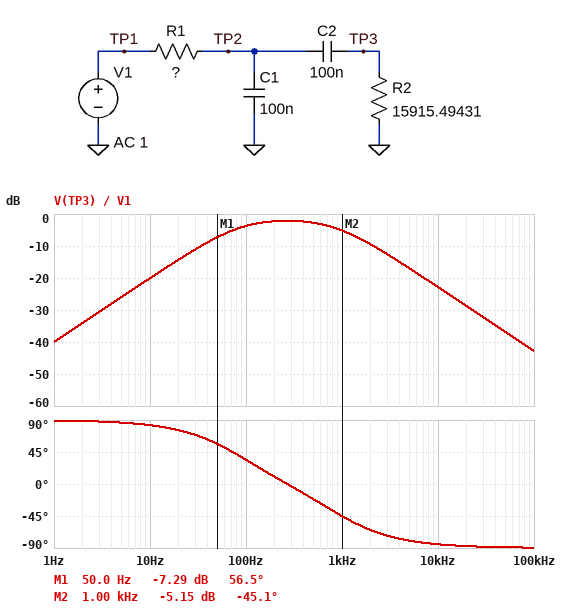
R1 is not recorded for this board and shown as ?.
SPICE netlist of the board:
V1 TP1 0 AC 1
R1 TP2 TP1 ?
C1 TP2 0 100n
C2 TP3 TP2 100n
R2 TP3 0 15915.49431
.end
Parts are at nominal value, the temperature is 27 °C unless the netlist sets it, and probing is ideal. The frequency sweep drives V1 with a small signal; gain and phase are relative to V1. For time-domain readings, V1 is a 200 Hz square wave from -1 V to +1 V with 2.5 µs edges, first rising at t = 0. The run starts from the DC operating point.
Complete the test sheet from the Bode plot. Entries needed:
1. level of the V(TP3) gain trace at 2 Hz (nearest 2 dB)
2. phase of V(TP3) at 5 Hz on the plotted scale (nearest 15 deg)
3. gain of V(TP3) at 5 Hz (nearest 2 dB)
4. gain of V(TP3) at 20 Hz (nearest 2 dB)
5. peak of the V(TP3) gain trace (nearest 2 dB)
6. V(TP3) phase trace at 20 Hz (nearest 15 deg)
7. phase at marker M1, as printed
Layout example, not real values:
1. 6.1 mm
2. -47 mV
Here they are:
1. -34 dB
2. 90 deg
3. -26 dB
4. -14 dB
5. -2 dB
6. 75 deg
7. 56.5 deg
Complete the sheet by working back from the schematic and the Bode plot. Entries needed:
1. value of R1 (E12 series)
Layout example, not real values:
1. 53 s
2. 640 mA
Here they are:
1. 2.2 kΩ
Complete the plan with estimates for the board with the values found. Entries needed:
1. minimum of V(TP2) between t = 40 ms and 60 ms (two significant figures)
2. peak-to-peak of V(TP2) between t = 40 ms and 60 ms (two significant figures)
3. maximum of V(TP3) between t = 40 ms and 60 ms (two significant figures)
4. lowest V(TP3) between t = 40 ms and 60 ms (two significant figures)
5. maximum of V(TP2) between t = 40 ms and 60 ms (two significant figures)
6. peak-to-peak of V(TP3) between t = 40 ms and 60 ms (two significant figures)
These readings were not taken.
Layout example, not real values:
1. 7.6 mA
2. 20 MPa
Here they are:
1. -940 mV
2. 1.9 V
3. 1.0 V
4. -1.0 V
5. 940 mV
6. 2.1 V
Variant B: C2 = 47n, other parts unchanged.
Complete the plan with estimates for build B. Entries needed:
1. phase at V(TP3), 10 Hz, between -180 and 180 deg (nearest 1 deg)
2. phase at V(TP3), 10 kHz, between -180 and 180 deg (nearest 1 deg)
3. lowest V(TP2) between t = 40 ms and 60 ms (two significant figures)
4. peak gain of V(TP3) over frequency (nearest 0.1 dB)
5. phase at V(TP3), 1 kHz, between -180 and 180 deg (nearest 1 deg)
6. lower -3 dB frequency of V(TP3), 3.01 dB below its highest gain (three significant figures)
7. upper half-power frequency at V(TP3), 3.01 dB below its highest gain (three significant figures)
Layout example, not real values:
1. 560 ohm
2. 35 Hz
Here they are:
1. 86 deg
2. -84 deg
3. -980 mV
4. -3.1 dB
5. -39 deg
6. 132 Hz
7. 1.17 kHz
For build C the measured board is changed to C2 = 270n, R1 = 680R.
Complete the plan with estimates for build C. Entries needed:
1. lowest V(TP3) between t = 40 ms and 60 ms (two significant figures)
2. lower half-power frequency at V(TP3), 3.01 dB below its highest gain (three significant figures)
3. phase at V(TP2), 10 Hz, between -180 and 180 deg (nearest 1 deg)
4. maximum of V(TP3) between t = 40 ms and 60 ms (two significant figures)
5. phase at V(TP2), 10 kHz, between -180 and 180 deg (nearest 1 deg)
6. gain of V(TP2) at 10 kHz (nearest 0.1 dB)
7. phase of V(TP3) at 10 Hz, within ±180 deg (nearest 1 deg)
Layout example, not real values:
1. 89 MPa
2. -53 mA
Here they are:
1. -1.1 V
2. 34.5 Hz
3. -1 deg
4. 1.1 V
5. -76 deg
6. -12.9 dB
7. 74 deg
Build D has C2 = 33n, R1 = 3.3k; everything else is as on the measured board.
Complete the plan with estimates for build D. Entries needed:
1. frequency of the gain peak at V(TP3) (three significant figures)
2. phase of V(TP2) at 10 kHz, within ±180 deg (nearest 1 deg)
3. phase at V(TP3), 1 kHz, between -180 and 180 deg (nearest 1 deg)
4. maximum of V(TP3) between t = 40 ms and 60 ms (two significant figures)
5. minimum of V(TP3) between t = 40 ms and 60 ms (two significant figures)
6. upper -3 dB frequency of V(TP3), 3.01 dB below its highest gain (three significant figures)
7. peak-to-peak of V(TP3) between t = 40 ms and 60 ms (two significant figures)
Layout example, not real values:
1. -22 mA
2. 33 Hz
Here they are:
1. 382 Hz
2. -87 deg
3. -44 deg
4. 800 mV
5. -800 mV
6. 1.03 kHz
7. 1.6 V
